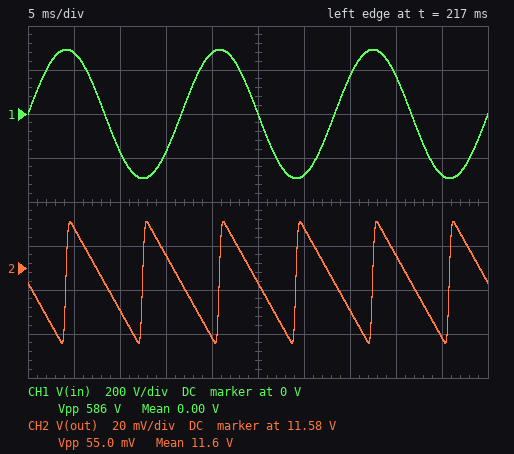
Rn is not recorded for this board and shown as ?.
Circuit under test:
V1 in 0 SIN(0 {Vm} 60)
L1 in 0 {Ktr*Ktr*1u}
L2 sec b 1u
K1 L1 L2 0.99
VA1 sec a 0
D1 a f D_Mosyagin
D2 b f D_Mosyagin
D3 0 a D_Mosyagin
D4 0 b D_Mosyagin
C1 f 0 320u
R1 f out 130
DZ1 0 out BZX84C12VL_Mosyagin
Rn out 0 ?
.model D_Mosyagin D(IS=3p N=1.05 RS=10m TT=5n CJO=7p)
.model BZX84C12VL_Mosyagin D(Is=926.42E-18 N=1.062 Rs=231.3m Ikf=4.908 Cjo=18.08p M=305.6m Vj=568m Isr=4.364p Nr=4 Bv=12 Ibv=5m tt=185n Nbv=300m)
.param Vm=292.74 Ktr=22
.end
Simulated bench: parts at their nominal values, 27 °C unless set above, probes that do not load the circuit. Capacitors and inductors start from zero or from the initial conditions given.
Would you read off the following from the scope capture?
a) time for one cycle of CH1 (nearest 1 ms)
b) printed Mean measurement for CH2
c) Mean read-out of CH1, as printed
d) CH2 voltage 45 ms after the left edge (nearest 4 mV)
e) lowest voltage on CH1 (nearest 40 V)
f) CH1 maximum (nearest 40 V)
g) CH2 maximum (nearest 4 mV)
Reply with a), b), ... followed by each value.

a) 17 ms
b) 11.6 V
c) 0.00 V
d) 11.548 V
e) -280 V
f) 280 V
g) 11.600 V
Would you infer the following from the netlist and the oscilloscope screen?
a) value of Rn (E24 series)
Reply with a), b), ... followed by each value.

a) 4.7 kΩ
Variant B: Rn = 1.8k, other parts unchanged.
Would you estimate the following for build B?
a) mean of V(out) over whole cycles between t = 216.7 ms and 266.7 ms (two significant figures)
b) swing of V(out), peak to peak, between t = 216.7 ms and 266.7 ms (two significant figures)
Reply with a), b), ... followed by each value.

a) 11 V
b) 130 mV
